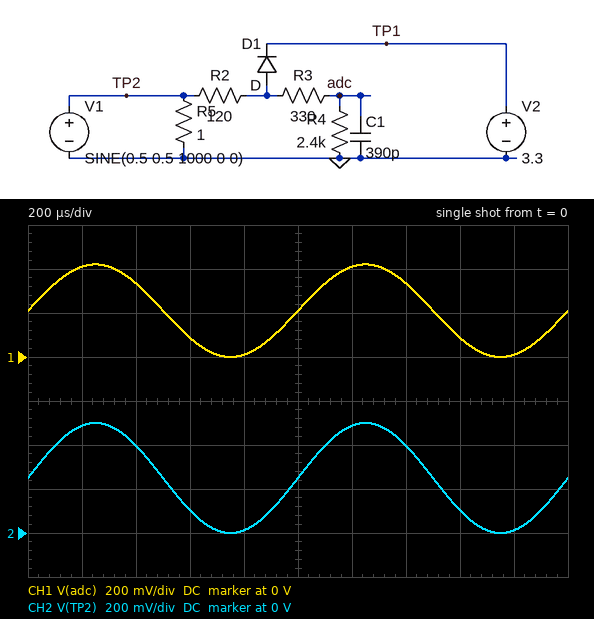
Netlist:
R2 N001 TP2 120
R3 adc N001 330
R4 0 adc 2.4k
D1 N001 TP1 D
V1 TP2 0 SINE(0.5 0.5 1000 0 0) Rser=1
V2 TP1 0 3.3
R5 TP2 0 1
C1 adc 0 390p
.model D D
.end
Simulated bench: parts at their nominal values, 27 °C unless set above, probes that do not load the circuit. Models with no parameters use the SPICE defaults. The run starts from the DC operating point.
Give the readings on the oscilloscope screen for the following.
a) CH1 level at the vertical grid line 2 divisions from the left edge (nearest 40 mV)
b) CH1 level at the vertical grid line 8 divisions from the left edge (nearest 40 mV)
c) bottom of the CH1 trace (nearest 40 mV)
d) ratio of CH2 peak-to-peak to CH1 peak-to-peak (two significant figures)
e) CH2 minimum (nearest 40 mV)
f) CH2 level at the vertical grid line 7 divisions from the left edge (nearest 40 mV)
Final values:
320 mV
80 mV
0 V
1.2
0 V
400 mV
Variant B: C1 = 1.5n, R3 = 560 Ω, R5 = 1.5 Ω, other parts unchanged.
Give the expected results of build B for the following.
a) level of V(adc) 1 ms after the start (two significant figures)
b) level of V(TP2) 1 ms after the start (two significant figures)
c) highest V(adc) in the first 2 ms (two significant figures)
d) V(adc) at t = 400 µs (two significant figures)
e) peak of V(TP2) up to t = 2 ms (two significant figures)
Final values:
230 mV
300 mV
470 mV
370 mV
600 mV
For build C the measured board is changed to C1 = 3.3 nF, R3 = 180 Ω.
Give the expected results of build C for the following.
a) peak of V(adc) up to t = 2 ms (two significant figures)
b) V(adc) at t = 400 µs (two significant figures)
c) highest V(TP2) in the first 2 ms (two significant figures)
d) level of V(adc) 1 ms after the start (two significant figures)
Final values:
440 mV
350 mV
500 mV
220 mV
